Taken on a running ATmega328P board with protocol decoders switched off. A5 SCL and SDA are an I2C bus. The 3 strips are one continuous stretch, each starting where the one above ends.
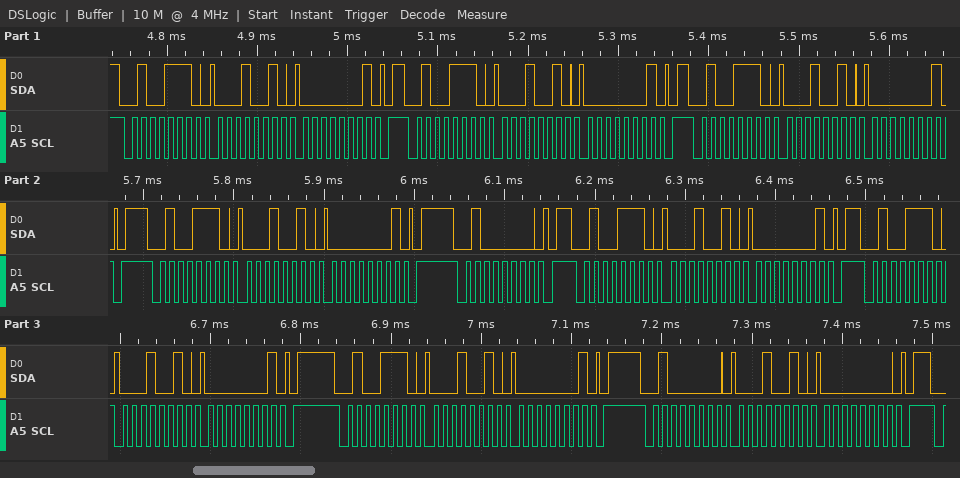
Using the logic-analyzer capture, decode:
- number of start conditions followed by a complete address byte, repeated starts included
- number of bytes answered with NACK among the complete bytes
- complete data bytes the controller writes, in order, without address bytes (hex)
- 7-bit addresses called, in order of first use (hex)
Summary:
9
0
12 01 12 01 12 01 12 01 12 01 12 01 12 01 12 00
0x27 0x20
